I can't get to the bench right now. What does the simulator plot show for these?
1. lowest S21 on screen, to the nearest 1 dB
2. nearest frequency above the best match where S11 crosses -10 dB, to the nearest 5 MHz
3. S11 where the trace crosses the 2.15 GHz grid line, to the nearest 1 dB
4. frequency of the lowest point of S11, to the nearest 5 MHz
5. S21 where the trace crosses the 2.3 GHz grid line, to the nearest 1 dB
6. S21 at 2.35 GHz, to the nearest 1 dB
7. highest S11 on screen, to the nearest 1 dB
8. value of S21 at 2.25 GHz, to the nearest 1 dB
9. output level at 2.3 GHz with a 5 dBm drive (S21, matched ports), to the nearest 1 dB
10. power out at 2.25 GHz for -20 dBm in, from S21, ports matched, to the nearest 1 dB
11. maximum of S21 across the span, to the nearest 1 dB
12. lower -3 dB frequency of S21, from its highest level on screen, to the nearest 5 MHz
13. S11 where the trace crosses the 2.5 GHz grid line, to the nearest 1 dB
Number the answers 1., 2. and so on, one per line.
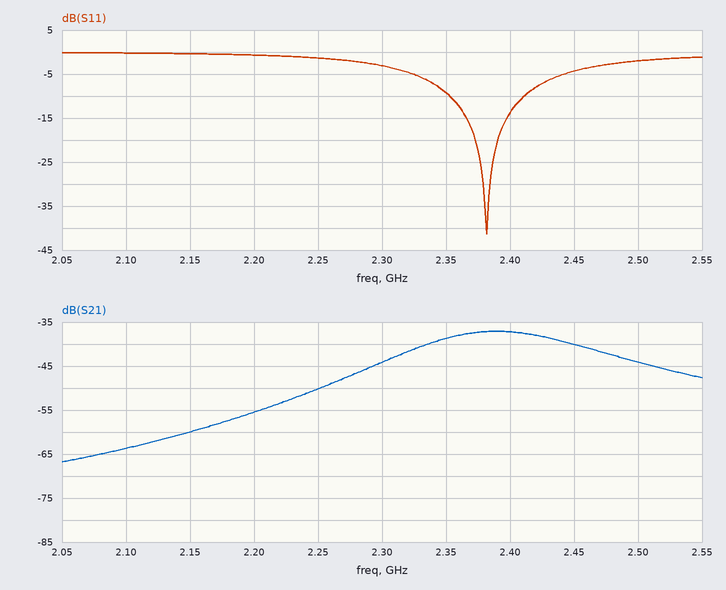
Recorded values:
1. -67 dB
2. 2.410 GHz
3. 0 dB
4. 2.380 GHz
5. -44 dB
6. -39 dB
7. 0 dB
8. -50 dB
9. -39 dBm
10. -70 dBm
11. -37 dB
12. 2.335 GHz
13. -2 dB
